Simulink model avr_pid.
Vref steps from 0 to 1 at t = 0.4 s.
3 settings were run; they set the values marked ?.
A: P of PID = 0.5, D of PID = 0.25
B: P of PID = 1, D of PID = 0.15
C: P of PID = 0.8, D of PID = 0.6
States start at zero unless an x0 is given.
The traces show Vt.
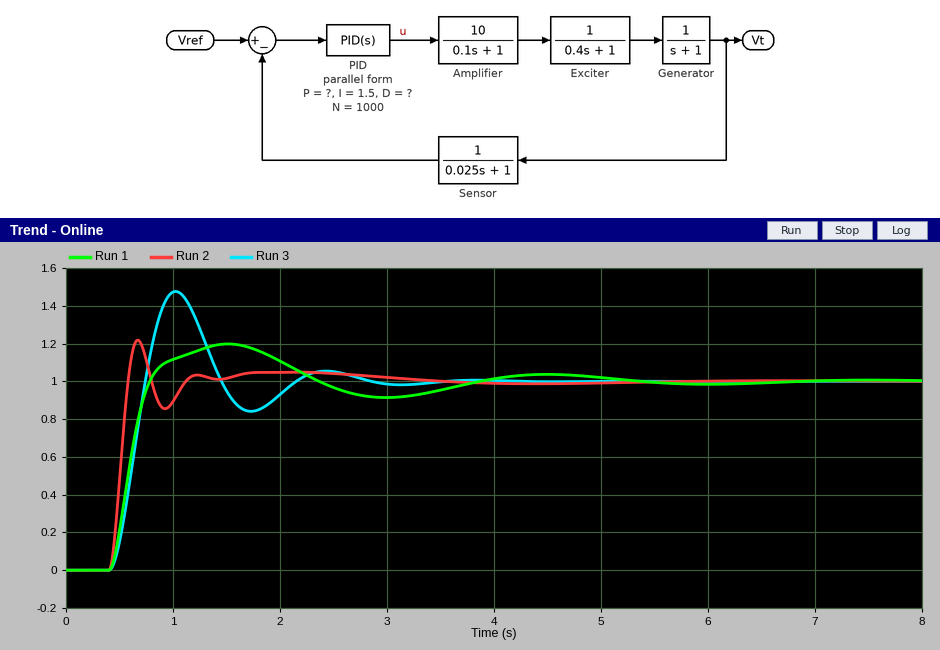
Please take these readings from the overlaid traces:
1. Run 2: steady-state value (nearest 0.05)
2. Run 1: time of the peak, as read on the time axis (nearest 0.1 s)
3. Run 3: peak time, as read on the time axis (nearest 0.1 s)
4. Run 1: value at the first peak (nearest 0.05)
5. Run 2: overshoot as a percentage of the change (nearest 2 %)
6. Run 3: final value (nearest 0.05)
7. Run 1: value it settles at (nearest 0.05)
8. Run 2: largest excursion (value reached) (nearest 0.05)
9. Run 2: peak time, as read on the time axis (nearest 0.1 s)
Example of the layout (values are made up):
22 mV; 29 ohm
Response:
1.00; 1.5 s; 1.0 s; 1.20; 22 %; 1.00; 1.00; 1.20; 0.7 s
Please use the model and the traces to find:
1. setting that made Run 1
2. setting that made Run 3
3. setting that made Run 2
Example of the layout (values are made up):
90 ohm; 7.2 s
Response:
A; B; C
